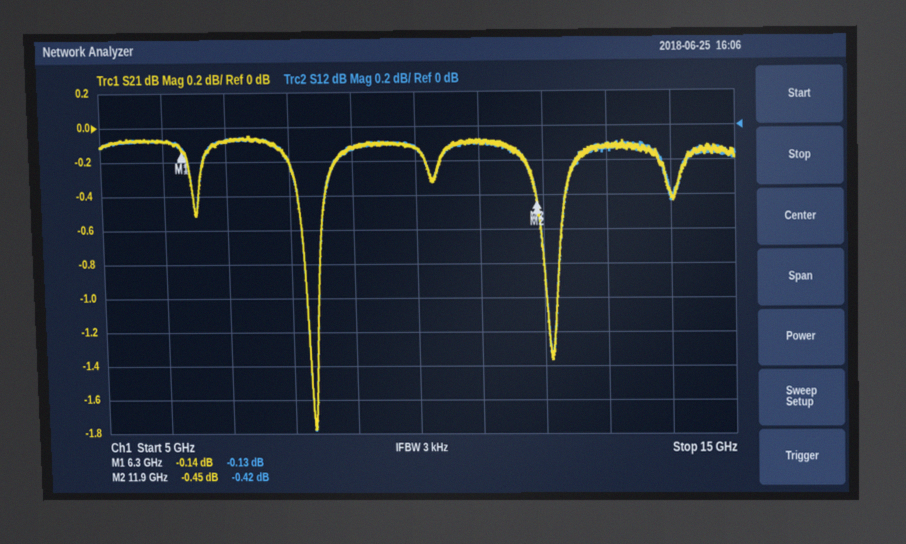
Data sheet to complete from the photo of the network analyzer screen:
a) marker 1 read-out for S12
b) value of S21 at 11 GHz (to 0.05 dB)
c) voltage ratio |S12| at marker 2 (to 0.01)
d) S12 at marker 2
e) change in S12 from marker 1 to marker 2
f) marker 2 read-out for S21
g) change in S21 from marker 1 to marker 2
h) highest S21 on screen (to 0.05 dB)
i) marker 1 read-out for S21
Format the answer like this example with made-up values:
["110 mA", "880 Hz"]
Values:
["-0.13 dB", "-0.10 dB", "0.95", "-0.42 dB", "-0.29 dB", "-0.45 dB", "-0.31 dB", "-0.05 dB", "-0.14 dB"]
